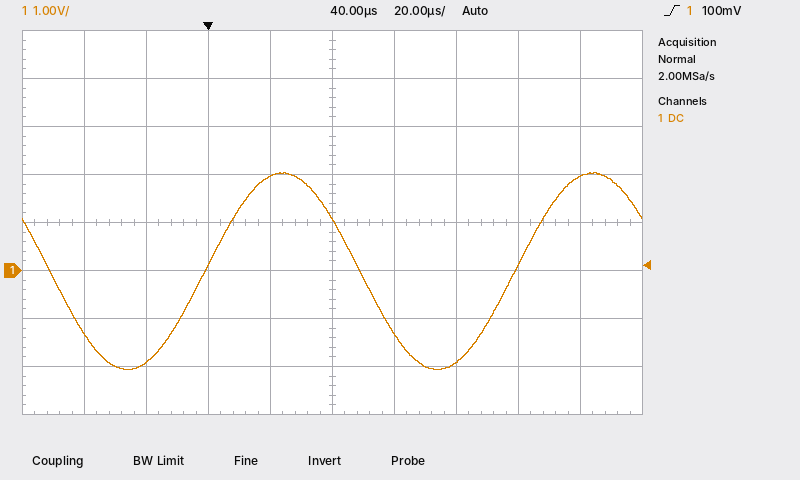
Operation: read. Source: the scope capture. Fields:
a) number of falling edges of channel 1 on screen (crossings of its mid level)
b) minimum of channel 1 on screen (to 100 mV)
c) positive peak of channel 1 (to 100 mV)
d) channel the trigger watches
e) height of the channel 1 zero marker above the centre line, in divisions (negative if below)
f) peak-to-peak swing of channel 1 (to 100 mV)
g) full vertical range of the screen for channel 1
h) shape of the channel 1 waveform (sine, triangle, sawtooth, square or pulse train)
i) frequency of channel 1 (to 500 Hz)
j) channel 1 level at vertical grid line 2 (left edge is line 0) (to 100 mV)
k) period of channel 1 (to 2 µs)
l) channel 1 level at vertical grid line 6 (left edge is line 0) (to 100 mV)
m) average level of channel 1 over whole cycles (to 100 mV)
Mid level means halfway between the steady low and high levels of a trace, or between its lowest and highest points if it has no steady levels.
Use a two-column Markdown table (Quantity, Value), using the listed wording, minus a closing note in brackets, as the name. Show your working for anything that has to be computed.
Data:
| Quantity | Value |
|---|---|
| number of falling edges of channel 1 on screen | 2 |
| minimum of channel 1 on screen | -2.1 V |
| positive peak of channel 1 | 2.0 V |
| channel the trigger watches | channel 1 |
| height of the channel 1 zero marker above the centre line, in divisions | -1.0 div |
| peak-to-peak swing of channel 1 | 2.0 V − (-2.1 V) = 4.1 V |
| full vertical range of the screen for channel 1 | 8 V |
| shape of the channel 1 waveform | sine |
| frequency of channel 1 | 1 / 100 µs ≈ 10.0 kHz |
| channel 1 level at vertical grid line 2 (left edge is line 0) | -1.9 V |
| period of channel 1 | 100 µs |
| channel 1 level at vertical grid line 6 (left edge is line 0) | -1.3 V |
| average level of channel 1 over whole cycles | (2.0 V + (-2.1 V)) / 2 ≈ 0.0 V |
